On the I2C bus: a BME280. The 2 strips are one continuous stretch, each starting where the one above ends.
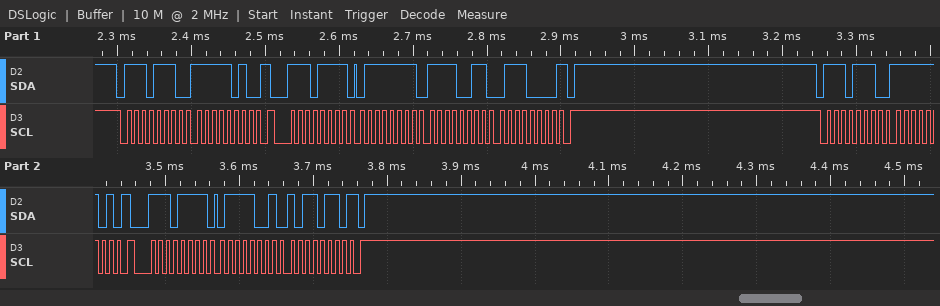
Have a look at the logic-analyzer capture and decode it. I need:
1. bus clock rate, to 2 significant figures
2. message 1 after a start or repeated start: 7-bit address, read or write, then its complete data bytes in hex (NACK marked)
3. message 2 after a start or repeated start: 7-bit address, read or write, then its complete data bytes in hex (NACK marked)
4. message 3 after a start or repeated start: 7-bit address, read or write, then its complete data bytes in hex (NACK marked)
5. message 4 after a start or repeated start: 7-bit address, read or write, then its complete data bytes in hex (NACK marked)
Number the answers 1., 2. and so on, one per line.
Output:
1. 100 kHz
2. 0x77 write: FA
3. 0x77 read: 7F F3 70 NACK
4. 0x77 write: FD
5. 0x77 read: 79 B6 NACK
